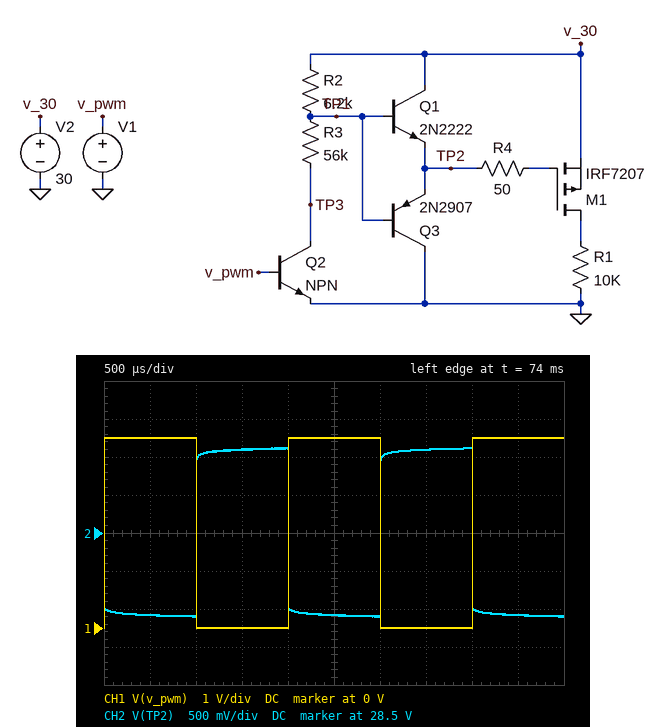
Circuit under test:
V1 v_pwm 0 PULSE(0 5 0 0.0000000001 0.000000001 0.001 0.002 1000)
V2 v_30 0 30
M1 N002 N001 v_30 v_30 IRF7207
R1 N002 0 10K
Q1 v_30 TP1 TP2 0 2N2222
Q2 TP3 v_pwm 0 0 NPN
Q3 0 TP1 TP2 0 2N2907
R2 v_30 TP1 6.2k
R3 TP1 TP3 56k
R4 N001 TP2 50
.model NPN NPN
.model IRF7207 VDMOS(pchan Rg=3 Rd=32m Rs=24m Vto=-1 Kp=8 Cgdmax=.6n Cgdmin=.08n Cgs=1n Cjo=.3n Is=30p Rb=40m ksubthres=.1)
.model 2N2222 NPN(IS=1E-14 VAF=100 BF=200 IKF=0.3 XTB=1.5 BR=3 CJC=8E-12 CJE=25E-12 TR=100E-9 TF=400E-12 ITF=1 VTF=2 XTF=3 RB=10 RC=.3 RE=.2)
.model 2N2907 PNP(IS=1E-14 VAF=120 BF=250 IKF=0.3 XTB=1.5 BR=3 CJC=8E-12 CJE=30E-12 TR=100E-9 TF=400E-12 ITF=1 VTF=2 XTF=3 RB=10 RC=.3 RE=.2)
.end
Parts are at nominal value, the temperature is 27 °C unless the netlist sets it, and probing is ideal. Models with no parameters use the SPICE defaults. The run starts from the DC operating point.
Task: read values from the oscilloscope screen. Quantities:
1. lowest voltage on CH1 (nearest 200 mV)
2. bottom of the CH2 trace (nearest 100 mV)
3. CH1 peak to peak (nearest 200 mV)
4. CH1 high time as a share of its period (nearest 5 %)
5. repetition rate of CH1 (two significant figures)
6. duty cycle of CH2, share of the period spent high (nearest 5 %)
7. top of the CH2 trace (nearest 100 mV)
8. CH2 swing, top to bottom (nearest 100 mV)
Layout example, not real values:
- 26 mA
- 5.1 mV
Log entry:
- 0 V
- 27.4 V
- 5.0 V
- 50 %
- 500 Hz
- 50 %
- 29.6 V
- 2.2 V
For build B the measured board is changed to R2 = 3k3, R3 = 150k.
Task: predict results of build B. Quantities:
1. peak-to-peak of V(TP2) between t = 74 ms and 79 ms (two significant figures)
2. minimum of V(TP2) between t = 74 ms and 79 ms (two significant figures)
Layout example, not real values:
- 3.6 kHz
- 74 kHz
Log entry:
- 33 mV
- 30 V
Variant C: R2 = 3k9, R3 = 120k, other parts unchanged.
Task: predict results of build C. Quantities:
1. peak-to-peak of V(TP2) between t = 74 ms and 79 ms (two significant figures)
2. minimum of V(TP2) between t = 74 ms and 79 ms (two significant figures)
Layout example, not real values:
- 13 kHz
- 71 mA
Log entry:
- 180 mV
- 29 V
